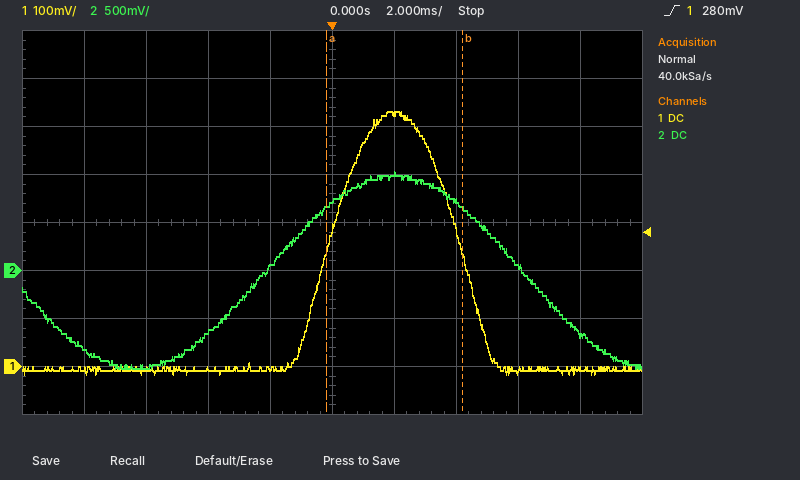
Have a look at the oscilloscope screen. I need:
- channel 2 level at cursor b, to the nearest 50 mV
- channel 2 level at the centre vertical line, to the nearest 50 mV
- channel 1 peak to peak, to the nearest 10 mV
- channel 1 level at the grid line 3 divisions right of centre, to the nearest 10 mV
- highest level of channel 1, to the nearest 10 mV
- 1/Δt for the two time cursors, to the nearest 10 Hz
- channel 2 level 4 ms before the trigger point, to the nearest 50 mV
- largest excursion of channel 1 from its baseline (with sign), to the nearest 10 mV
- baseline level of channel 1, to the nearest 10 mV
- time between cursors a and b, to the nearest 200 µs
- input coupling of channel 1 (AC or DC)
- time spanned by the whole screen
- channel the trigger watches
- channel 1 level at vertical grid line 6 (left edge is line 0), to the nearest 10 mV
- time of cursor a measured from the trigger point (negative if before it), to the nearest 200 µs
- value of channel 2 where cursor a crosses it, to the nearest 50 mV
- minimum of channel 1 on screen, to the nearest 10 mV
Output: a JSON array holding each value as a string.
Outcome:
["650 mV", "700 mV", "550 mV", "-10 mV", "530 mV", "230 Hz", "-650 mV", "+540 mV", "-10 mV", "4.4 ms", "DC", "20 ms", "channel 1", "530 mV", "-200 µs", "650 mV", "-20 mV"]
